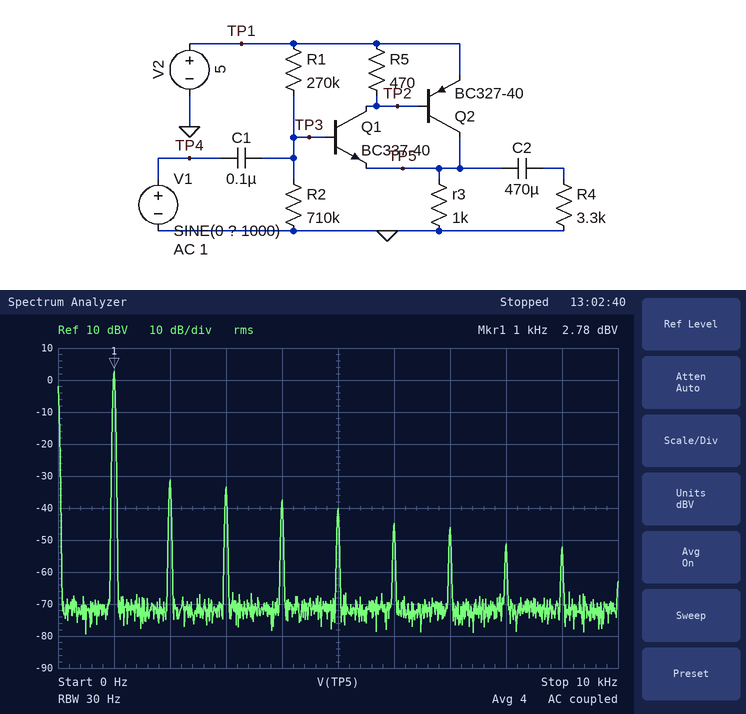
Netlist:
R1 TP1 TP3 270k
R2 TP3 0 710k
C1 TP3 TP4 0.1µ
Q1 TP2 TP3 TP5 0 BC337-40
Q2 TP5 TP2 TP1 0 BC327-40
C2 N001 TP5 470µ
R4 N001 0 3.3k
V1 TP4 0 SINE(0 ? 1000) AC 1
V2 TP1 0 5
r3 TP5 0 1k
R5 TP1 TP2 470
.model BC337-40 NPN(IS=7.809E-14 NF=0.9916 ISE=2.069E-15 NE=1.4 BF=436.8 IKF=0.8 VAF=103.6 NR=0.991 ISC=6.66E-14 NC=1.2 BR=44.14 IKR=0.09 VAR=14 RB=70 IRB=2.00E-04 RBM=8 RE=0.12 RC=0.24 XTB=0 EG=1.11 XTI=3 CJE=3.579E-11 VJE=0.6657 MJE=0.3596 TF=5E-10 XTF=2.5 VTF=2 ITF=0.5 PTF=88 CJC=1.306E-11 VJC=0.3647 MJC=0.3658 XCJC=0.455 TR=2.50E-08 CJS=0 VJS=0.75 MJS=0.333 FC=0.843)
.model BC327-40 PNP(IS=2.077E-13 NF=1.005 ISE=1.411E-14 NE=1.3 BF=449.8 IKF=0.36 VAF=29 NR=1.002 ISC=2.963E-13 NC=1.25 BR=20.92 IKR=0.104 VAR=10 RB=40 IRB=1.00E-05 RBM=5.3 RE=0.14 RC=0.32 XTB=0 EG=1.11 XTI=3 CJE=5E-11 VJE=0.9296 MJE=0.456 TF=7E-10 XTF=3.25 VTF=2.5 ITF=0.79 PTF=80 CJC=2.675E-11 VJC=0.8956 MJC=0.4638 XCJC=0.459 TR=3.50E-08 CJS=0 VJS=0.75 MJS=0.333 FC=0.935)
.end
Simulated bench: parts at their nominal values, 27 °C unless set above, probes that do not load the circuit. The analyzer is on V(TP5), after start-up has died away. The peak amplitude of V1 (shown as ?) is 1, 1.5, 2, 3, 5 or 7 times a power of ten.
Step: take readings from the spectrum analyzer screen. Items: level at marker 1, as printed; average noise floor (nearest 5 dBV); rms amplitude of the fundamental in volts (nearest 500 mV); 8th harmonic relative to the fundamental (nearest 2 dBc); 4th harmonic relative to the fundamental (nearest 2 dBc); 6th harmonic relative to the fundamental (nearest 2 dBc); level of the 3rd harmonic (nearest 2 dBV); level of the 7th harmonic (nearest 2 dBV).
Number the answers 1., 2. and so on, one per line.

1. 2.78 dBV
2. -70 dBV
3. 1.5 V
4. -54 dBc
5. -40 dBc
6. -48 dBc
7. -34 dBV
8. -46 dBV
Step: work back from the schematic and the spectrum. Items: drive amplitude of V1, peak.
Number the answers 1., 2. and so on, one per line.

1. 2 V
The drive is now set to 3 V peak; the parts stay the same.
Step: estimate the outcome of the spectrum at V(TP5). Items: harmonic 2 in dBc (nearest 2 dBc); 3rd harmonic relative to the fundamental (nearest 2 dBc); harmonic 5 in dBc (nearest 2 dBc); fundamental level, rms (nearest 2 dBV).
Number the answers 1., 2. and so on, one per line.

1. -12 dBc
2. -22 dBc
3. -30 dBc
4. 4 dBV
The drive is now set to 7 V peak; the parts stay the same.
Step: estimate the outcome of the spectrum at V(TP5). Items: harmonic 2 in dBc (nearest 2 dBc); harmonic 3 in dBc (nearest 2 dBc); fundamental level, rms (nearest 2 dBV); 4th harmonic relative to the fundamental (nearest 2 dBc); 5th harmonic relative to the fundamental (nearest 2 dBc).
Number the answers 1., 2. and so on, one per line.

1. -4 dBc
2. -12 dBc
3. 2 dBV
4. -38 dBc
5. -20 dBc
